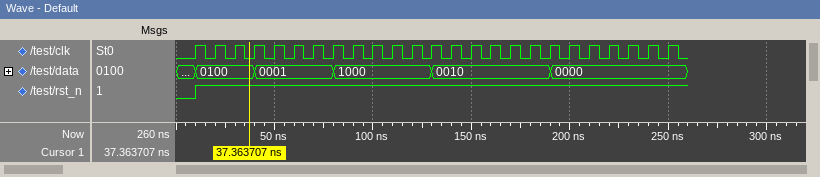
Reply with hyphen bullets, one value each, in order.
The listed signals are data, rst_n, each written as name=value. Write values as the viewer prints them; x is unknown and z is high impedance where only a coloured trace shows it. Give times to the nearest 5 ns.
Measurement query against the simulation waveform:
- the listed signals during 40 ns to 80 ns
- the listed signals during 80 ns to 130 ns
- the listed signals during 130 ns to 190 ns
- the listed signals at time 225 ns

- data=0001, rst_n=1
- data=1000, rst_n=1
- data=0010, rst_n=1
- data=0000, rst_n=1
